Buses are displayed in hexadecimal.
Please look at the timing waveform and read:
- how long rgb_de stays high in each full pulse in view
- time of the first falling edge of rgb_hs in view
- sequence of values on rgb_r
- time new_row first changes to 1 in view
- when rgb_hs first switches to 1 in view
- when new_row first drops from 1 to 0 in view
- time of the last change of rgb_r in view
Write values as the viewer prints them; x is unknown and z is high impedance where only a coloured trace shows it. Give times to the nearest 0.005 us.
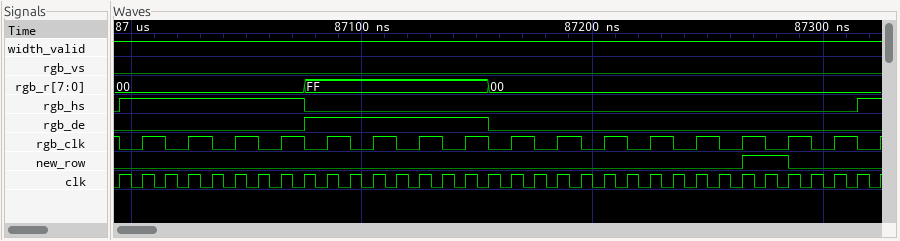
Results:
0.08 us
87.075 us
00, FF, 00
87.265 us
86.995 us
87.285 us
87.155 us
